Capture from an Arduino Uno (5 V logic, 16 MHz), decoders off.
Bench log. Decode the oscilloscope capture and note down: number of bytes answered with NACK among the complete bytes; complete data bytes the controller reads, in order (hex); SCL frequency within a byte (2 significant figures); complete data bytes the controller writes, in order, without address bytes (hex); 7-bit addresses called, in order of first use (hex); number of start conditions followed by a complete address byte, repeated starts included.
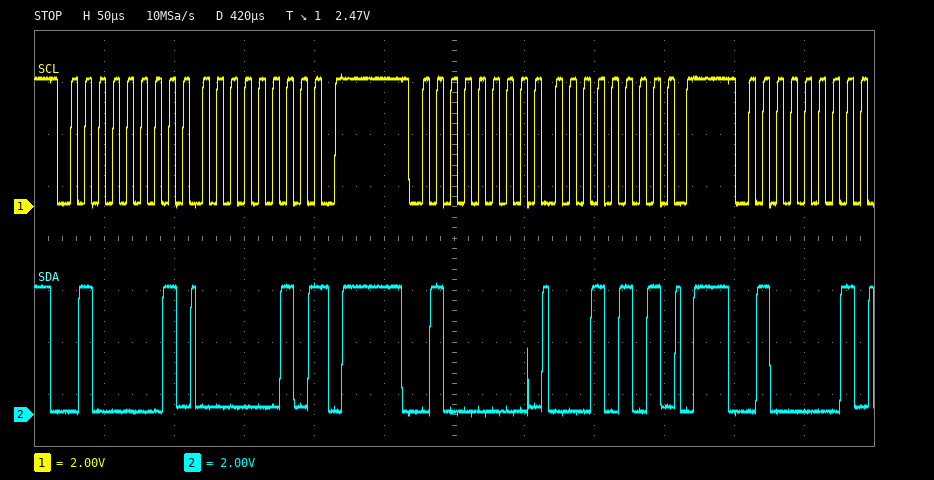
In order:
1
02
100 kHz
15
0x20
3
